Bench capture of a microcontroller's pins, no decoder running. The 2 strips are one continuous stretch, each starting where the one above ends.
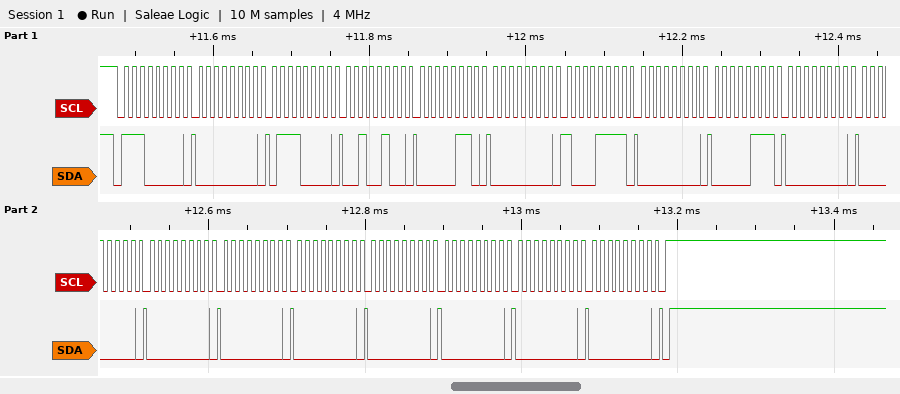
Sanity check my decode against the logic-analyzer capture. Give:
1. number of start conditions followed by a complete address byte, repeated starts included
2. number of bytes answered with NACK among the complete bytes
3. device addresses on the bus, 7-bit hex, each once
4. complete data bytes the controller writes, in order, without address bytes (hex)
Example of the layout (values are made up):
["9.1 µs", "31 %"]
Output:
["1", "0", "0x70", "00 70 24 06 00 8F 00 07 00 00 00 00 00 00 00 00 00"]
